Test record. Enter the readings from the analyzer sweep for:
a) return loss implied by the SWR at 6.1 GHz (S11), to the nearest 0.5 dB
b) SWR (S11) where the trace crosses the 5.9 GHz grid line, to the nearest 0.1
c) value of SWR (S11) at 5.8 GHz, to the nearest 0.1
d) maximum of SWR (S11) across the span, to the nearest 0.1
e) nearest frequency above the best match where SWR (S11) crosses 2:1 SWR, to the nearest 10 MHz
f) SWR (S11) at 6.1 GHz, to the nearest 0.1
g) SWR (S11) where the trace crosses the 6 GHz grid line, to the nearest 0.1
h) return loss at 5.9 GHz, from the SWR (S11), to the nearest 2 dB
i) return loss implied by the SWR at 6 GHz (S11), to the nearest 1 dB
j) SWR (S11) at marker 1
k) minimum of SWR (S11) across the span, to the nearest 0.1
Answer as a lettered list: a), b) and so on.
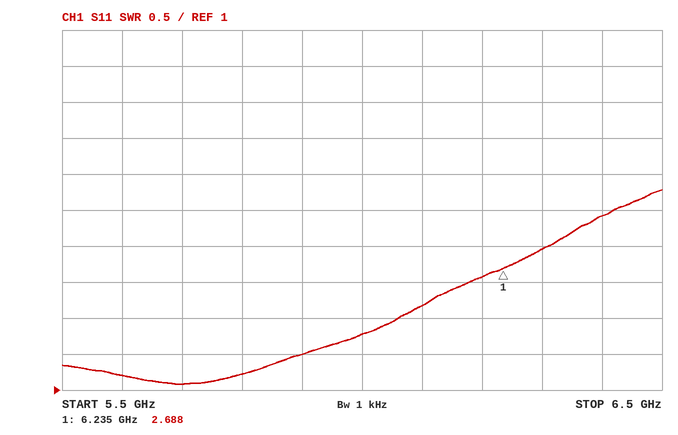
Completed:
a) 8.5 dB
b) 1.5
c) 1.2
d) 3.8
e) 6.06 GHz
f) 2.2
g) 1.8
h) 14 dB
i) 11 dB
j) 2.688
k) 1.1
